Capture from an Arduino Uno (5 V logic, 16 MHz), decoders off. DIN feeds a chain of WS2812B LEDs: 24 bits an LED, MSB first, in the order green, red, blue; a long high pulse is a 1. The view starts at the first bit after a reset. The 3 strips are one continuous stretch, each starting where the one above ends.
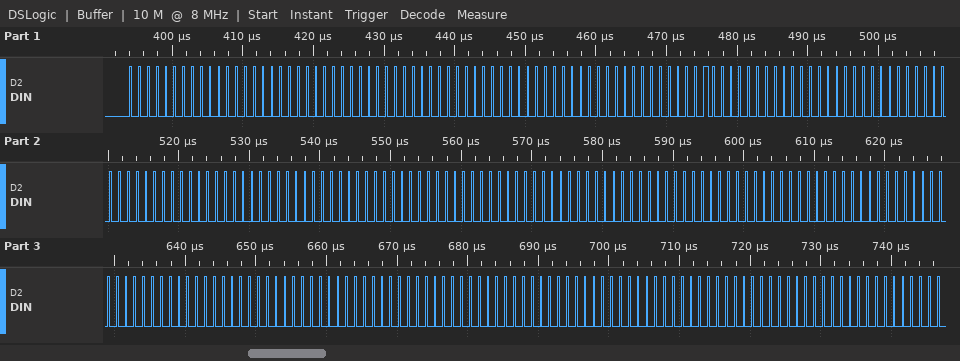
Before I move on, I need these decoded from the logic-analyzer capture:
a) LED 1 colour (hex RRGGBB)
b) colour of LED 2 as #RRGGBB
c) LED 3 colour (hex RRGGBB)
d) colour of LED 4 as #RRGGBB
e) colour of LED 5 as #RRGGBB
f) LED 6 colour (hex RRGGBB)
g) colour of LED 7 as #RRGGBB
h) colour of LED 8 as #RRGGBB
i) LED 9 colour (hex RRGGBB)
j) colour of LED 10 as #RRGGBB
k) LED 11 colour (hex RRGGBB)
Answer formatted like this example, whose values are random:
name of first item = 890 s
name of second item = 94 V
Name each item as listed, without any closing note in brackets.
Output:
LED 1 colour = #000000
colour of LED 2 as #RRGGBB = #000000
LED 3 colour = #000040
colour of LED 4 as #RRGGBB = #000000
colour of LED 5 as #RRGGBB = #000000
LED 6 colour = #000000
colour of LED 7 as #RRGGBB = #000000
colour of LED 8 as #RRGGBB = #000000
LED 9 colour = #000000
colour of LED 10 as #RRGGBB = #000000
LED 11 colour = #000000
